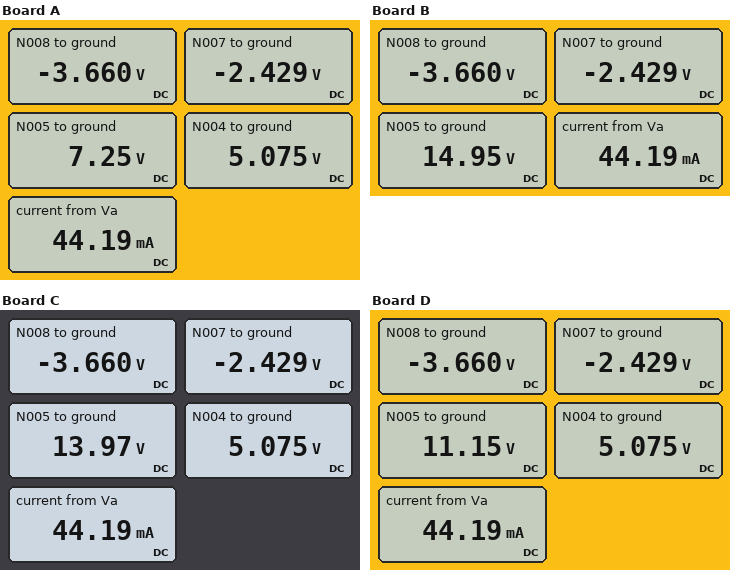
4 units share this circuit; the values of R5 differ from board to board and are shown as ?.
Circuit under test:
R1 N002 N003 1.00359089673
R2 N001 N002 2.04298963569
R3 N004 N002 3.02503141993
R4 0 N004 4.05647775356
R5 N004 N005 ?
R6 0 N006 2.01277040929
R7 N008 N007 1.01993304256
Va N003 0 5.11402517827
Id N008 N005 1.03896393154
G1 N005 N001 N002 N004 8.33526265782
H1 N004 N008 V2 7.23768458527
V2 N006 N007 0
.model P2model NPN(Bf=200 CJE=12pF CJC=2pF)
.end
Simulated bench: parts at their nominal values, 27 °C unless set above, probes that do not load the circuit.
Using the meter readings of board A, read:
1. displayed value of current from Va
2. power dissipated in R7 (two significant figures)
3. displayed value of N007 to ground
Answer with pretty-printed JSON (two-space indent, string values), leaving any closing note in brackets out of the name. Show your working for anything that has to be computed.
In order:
{
  "displayed value of current from Va": "44.19 mA",
  "power dissipated in R7": "(-2.429 V - (-3.66 V))^2 / 1.02 Ω = 1.5 W",
  "displayed value of N007 to ground": "-2.429 V"
}
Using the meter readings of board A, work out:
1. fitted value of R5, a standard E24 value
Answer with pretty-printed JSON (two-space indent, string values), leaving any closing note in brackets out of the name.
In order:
{
  "fitted value of R5, a standard E24 value": "2 Ω"
}
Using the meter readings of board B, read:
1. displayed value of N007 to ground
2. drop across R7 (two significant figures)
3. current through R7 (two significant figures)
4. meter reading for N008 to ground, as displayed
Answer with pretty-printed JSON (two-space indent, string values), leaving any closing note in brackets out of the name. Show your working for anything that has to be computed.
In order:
{
  "displayed value of N007 to ground": "-2.429 V",
  "drop across R7": "-2.429 V - (-3.66 V) = 1.2 V",
  "current through R7": "(-2.429 V - (-3.66 V)) / 1.02 Ω = 1.2 A",
  "meter reading for N008 to ground, as displayed": "-3.660 V"
}
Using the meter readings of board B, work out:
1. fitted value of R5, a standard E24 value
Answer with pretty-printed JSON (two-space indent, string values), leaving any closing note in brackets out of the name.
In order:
{
  "fitted value of R5, a standard E24 value": "9.1 Ω"
}
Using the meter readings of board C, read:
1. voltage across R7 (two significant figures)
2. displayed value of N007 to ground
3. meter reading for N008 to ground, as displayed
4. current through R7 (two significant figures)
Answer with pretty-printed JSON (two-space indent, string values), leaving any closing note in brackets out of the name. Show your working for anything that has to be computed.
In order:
{
  "voltage across R7": "-2.429 V - (-3.66 V) = 1.2 V",
  "displayed value of N007 to ground": "-2.429 V",
  "meter reading for N008 to ground, as displayed": "-3.660 V",
  "current through R7": "(-2.429 V - (-3.66 V)) / 1.02 Ω = 1.2 A"
}
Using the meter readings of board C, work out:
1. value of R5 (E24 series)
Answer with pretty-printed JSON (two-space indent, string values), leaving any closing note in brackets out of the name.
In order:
{
  "value of R5": "8.2 Ω"
}
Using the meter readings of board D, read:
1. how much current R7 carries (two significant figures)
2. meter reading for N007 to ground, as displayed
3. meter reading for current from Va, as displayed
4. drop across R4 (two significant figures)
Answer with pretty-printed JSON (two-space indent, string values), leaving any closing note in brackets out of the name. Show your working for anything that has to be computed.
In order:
{
  "how much current R7 carries": "(-2.429 V - (-3.66 V)) / 1.02 Ω = 1.2 A",
  "meter reading for N007 to ground, as displayed": "-2.429 V",
  "meter reading for current from Va, as displayed": "44.19 mA",
  "drop across R4": "5.075 V = 5.1 V"
}
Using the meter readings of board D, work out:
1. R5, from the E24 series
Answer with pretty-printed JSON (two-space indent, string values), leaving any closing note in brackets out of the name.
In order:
{
  "R5, from the E24 series": "5.6 Ω"
}
